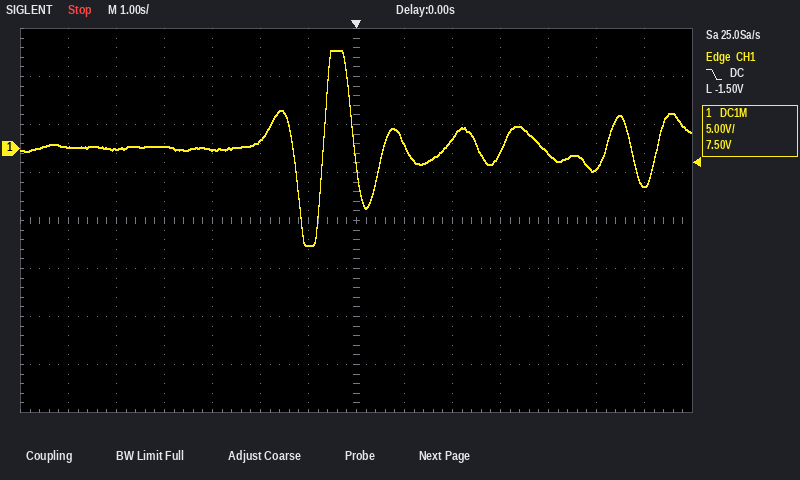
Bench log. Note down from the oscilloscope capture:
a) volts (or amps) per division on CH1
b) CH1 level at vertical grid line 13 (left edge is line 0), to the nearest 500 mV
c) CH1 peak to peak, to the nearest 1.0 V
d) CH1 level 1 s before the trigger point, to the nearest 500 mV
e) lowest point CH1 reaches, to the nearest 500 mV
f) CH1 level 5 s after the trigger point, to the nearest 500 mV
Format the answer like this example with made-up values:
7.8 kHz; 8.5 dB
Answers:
5 V; -4.0 V; 20.0 V; -10.0 V; -10.0 V; -2.0 V
